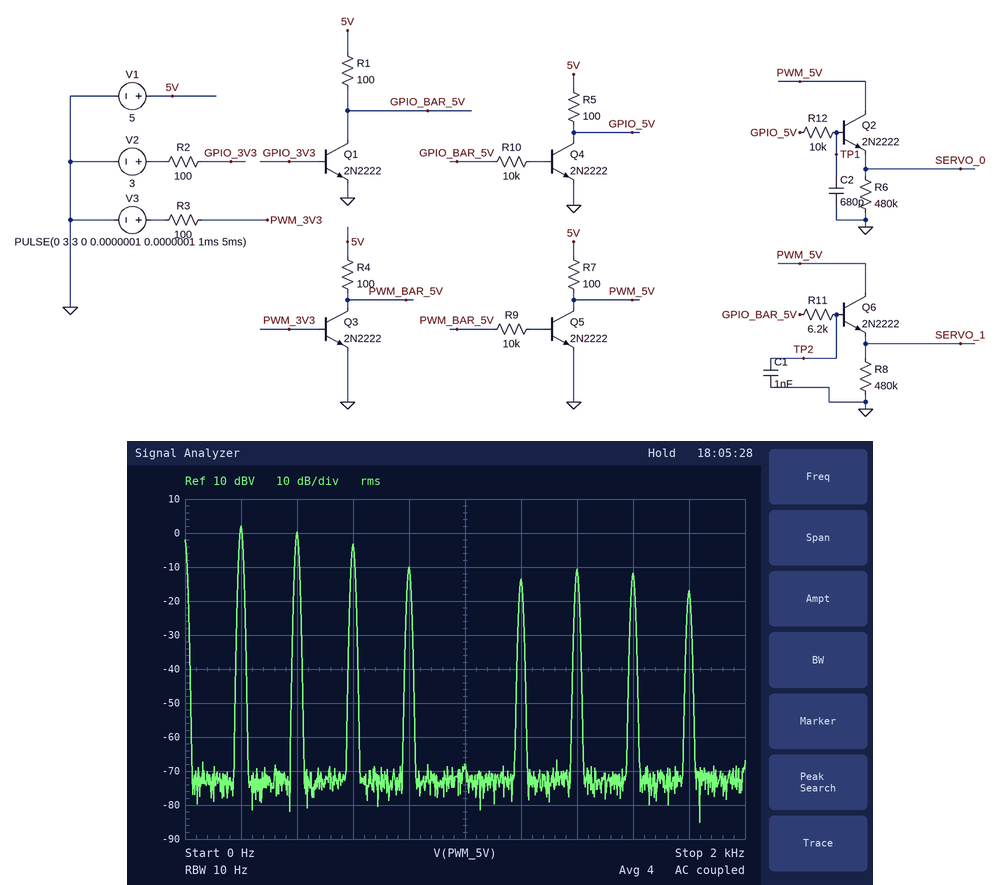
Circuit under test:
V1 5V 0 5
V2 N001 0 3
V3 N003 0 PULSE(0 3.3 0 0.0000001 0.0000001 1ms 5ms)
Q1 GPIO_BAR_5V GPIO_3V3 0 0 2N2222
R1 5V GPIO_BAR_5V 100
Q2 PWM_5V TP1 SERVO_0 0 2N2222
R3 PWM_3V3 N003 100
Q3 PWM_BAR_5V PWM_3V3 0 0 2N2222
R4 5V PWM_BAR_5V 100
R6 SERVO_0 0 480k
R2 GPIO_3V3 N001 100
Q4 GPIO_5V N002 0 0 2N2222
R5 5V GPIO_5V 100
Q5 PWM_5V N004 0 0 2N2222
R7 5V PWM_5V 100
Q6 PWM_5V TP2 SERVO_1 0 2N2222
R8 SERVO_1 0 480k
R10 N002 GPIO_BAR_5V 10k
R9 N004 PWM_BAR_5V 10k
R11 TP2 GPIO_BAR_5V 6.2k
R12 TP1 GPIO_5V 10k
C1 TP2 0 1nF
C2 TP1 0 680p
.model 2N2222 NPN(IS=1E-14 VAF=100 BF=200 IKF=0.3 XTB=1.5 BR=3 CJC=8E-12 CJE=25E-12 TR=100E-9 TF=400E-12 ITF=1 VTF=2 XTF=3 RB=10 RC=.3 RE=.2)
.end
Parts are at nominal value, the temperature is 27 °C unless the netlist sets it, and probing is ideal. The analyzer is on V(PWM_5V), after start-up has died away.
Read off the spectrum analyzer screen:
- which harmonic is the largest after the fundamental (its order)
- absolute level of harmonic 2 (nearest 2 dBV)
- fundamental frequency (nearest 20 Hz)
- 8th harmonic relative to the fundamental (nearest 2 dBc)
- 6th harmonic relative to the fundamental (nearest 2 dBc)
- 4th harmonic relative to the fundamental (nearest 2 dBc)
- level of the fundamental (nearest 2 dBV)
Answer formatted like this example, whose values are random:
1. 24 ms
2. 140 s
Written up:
1. 2
2. 0 dBV
3. 200 Hz
4. -14 dBc
5. -16 dBc
6. -12 dBc
7. 2 dBV
